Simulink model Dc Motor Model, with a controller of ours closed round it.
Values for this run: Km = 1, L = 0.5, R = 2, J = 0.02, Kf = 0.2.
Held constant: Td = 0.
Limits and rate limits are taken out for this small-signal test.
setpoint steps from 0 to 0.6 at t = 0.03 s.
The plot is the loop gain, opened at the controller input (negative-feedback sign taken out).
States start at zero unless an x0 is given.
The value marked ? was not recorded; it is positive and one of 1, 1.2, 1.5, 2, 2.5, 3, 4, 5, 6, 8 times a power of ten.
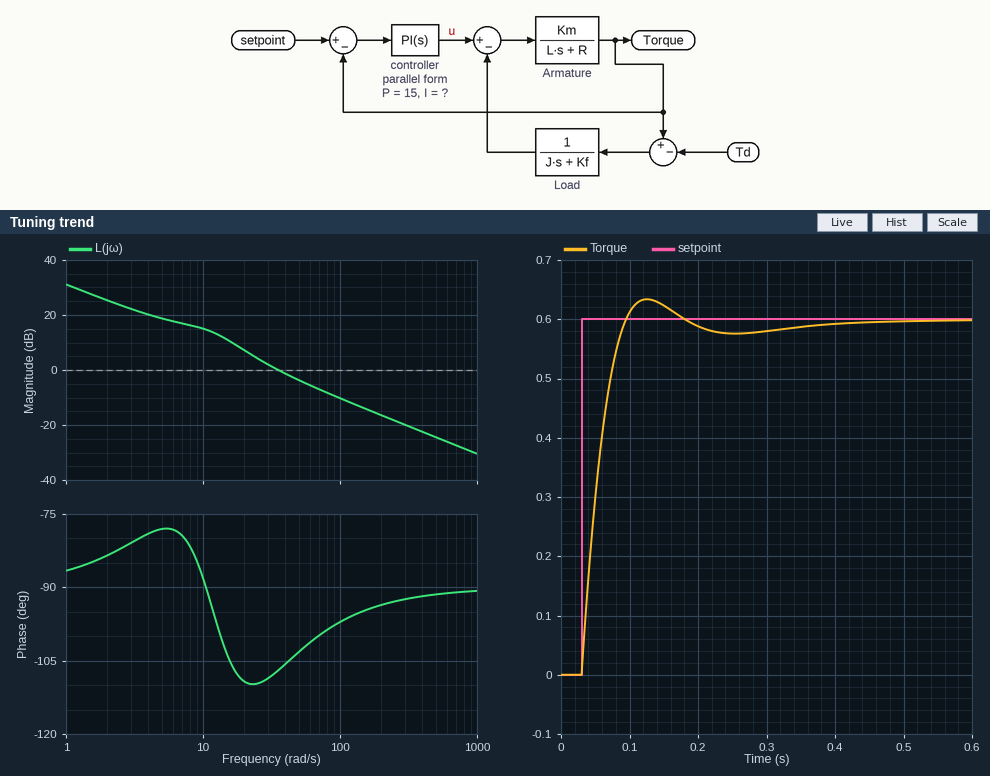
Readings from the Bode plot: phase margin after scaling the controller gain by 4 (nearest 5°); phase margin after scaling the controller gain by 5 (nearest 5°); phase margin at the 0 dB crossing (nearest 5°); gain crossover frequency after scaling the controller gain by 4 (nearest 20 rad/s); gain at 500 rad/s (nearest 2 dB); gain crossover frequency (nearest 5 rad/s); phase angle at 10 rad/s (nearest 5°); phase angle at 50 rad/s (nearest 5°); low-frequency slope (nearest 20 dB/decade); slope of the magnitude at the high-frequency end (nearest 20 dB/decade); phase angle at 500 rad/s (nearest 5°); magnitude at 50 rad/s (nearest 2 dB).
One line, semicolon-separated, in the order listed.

85°; 85°; 75°; 120 rad/s; -24 dB; 35 rad/s; -90°; -105°; -20 dB/decade; -20 dB/decade; -90°; -4 dB
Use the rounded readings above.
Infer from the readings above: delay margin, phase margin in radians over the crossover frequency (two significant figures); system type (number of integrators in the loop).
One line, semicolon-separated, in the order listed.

0.037 s; 1
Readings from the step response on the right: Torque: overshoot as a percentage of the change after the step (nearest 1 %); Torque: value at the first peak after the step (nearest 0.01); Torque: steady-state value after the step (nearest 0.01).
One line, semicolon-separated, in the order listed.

6 %; 0.63; 0.60
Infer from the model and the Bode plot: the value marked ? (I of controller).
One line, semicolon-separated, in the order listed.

250
